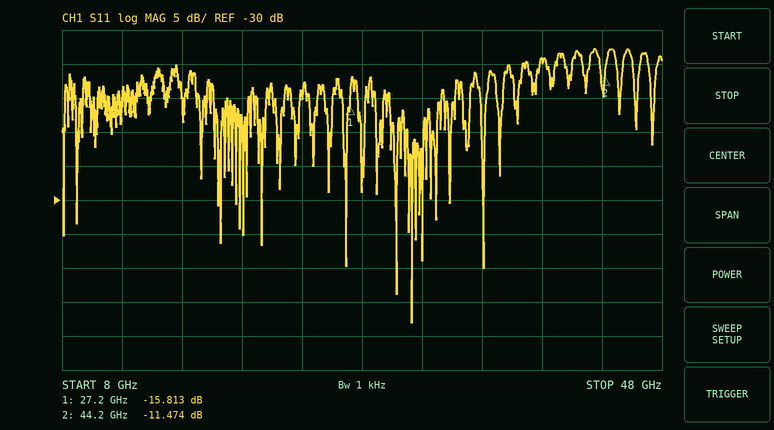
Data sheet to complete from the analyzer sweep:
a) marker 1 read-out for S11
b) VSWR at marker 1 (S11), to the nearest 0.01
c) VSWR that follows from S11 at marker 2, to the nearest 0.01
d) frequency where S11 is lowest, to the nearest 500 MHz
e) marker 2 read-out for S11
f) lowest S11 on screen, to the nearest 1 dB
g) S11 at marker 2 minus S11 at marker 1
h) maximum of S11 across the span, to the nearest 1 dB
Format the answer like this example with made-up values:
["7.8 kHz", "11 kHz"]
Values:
["-15.813 dB", "1.39", "1.73", "31.5 GHz", "-11.474 dB", "-48 dB", "4.339 dB", "-8 dB"]
